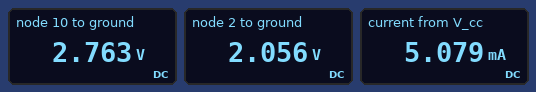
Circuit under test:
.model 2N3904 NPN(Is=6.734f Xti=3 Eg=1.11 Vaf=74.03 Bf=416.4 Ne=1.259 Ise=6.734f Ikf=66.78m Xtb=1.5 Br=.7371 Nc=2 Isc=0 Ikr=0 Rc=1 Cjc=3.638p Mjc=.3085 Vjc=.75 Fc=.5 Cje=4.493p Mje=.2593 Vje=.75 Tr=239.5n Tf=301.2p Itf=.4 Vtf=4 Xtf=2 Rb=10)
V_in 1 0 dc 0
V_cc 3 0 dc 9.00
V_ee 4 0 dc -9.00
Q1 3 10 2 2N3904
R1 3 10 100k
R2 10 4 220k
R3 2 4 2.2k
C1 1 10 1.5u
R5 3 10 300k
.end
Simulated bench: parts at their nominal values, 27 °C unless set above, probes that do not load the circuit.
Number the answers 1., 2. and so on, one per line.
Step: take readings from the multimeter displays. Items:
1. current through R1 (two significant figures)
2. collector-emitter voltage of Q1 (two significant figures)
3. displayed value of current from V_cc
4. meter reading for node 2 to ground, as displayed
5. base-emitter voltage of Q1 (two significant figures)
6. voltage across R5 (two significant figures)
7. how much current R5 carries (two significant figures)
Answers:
1. 62 µA
2. 6.9 V
3. 5.079 mA
4. 2.056 V
5. 710 mV
6. 6.2 V
7. 21 µA
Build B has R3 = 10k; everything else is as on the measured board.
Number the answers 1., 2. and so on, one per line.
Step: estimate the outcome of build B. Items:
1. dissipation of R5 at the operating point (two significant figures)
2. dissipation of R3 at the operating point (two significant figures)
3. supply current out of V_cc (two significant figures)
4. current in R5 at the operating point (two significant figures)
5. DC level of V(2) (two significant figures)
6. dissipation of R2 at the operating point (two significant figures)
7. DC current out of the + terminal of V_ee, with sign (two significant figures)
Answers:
1. 85 µW
2. 15 mW
3. 1.3 mA
4. 17 µA
5. 3.3 V
6. 760 µW
7. -1.3 mA
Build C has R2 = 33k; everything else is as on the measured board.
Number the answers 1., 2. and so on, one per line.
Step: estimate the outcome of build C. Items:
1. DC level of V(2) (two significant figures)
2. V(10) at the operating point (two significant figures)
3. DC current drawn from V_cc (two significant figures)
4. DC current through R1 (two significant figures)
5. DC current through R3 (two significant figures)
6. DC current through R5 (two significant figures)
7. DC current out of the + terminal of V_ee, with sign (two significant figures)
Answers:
1. -4.5 V
2. -3.8 V
3. 2.2 mA
4. 130 µA
5. 2.1 mA
6. 43 µA
7. -2.2 mA
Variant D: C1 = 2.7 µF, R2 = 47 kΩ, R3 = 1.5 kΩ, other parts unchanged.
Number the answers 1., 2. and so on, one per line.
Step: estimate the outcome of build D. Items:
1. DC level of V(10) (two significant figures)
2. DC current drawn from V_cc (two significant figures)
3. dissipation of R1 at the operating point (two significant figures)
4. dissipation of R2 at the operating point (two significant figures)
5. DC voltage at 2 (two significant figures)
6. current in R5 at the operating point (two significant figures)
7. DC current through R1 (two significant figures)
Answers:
1. -2.7 V
2. 3.9 mA
3. 1.4 mW
4. 850 µW
5. -3.4 V
6. 39 µA
7. 120 µA
